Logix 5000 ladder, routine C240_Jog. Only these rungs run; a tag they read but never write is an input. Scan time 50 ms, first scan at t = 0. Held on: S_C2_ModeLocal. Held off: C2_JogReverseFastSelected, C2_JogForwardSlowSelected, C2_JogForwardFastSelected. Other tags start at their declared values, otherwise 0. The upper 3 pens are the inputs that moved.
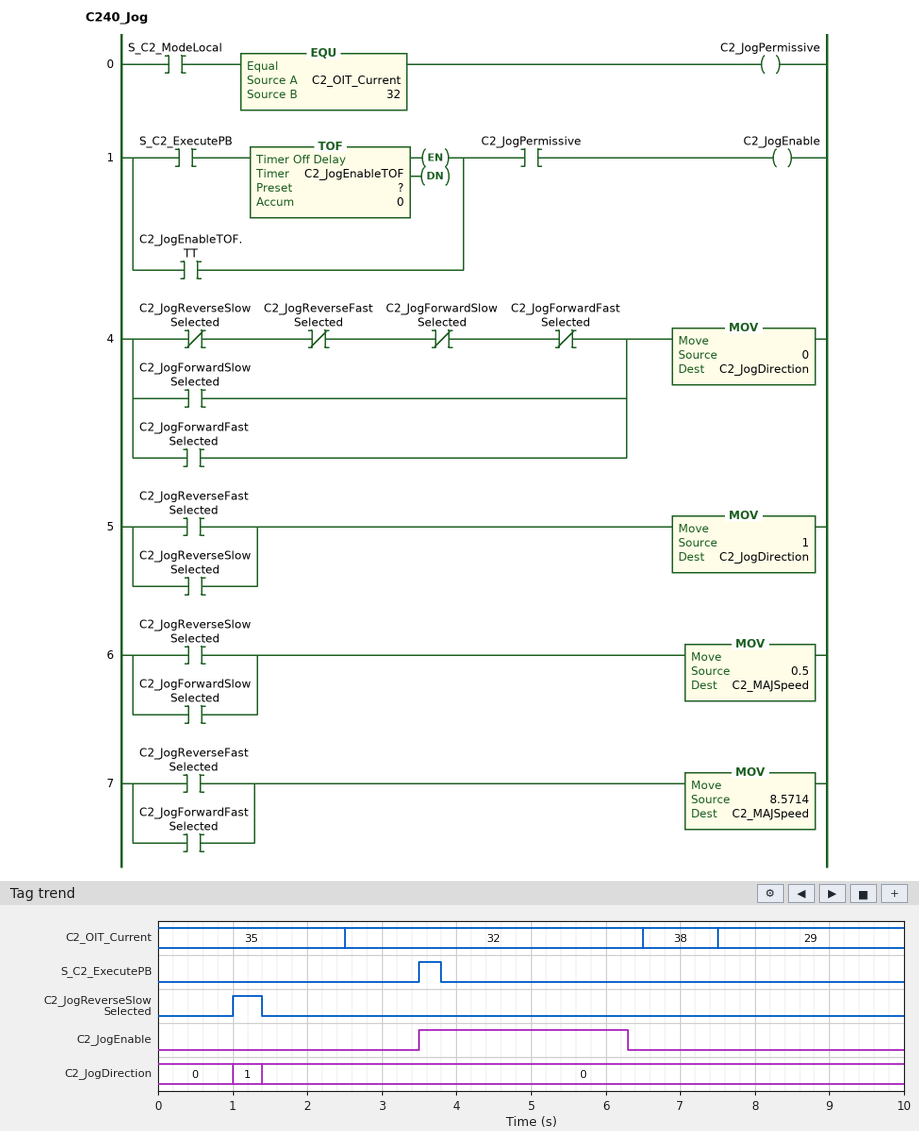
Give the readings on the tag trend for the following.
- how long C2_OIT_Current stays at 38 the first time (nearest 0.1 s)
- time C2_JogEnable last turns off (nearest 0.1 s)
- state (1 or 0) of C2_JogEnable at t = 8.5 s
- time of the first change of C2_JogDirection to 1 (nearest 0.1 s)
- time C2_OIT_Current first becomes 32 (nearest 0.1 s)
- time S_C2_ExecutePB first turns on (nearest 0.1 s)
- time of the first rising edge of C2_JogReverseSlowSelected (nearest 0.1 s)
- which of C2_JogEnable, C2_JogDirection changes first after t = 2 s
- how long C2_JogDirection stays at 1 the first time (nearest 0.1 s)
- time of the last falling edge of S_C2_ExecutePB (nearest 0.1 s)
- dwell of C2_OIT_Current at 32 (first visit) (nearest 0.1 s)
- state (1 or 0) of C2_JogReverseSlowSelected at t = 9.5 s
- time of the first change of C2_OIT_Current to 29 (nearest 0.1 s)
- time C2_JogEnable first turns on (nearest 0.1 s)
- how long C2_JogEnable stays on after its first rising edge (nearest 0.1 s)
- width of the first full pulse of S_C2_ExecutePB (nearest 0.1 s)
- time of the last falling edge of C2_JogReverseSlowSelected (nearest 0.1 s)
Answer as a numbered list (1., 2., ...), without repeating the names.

1. 1.0 s
2. 6.3 s
3. 0
4. 1.0 s
5. 2.5 s
6. 3.5 s
7. 1.0 s
8. C2_JogEnable
9. 0.4 s
10. 3.8 s
11. 4.0 s
12. 0
13. 7.5 s
14. 3.5 s
15. 2.8 s
16. 0.3 s
17. 1.4 s
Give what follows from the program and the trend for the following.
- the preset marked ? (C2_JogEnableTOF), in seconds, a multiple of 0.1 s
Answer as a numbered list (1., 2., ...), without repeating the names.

1. 2.5 s
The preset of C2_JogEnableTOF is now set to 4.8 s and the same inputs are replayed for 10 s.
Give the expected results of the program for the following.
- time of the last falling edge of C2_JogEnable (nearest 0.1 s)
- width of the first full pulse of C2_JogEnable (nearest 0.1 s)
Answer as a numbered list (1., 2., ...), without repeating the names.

1. 6.5 s
2. 3.0 s
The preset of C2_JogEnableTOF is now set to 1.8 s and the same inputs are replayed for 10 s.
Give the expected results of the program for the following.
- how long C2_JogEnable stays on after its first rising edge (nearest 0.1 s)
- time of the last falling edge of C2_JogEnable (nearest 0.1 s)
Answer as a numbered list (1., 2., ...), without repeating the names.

1. 2.1 s
2. 5.6 s
